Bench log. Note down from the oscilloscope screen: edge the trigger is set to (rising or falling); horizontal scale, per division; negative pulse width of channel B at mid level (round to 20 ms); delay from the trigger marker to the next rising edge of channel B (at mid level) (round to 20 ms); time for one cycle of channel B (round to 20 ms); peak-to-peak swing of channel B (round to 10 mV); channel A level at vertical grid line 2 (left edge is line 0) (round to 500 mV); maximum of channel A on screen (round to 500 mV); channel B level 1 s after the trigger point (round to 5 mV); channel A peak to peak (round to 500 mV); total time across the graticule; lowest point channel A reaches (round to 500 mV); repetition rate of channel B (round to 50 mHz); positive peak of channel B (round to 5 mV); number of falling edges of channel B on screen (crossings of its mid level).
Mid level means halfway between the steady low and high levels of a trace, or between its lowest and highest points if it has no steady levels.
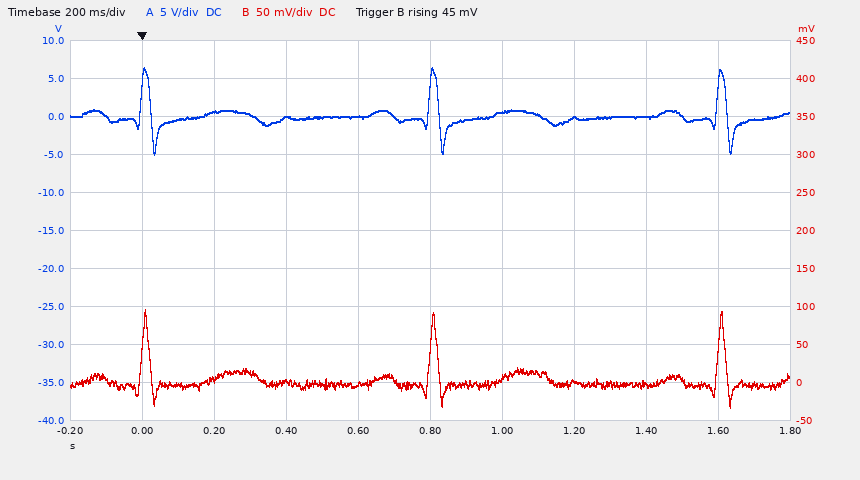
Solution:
rising
200 ms
780 ms
800 ms
800 ms
130 mV
500 mV
6.5 V
5 mV
11.5 V
2 s
-5.0 V
1.25 Hz
95 mV
3
